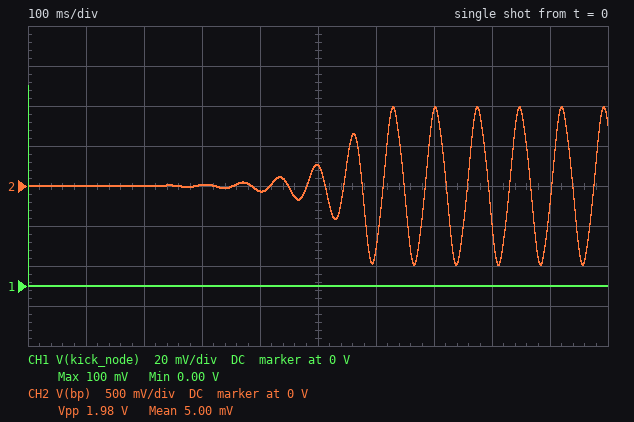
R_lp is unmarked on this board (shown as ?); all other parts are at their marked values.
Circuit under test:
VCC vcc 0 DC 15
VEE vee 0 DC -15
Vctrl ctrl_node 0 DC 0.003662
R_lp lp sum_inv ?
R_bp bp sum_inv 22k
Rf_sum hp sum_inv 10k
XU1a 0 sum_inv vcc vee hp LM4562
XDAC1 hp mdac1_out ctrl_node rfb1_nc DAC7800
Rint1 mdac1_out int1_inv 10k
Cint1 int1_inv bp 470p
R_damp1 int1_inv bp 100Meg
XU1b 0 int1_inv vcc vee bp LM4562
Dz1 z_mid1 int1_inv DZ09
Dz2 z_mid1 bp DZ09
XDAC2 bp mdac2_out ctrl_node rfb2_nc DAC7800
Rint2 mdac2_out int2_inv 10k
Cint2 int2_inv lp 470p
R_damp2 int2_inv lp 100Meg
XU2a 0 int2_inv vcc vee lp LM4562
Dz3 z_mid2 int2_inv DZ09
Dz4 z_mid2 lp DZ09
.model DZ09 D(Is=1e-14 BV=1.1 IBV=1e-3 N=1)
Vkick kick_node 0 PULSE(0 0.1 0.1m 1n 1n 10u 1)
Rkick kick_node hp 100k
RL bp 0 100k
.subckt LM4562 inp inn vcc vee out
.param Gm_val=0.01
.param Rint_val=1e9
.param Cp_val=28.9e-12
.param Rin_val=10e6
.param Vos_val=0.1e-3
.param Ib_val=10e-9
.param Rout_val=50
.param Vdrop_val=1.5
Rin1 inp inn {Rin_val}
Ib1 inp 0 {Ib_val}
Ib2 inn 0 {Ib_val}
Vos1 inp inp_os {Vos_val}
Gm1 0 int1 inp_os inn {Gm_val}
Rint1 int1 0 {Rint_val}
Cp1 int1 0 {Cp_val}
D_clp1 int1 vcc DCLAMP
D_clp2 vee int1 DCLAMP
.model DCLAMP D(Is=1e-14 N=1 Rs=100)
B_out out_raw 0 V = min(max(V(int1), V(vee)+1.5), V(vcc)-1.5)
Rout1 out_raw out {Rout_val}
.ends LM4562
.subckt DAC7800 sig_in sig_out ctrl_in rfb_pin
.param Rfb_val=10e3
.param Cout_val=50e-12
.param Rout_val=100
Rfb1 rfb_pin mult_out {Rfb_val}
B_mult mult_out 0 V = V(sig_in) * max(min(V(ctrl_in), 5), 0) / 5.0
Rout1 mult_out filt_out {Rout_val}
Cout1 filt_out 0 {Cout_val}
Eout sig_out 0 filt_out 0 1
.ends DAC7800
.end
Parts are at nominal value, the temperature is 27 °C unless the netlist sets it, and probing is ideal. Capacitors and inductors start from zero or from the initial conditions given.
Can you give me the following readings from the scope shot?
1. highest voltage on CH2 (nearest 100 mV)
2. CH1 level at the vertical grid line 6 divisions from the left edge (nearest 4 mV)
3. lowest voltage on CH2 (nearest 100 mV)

1.0 V
0 V
-1.0 V
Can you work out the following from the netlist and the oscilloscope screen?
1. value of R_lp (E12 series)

22 kΩ
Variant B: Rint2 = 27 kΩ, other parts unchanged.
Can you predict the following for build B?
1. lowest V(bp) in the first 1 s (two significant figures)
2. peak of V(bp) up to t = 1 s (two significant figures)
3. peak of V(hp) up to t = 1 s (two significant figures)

-1.2 V
1.2 V
480 mV
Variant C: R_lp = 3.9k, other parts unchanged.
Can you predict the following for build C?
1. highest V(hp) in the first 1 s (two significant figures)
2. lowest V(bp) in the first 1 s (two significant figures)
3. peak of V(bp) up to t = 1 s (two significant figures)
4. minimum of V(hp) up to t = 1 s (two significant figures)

2.1 V
-1.2 V
1.2 V
-2.1 V
